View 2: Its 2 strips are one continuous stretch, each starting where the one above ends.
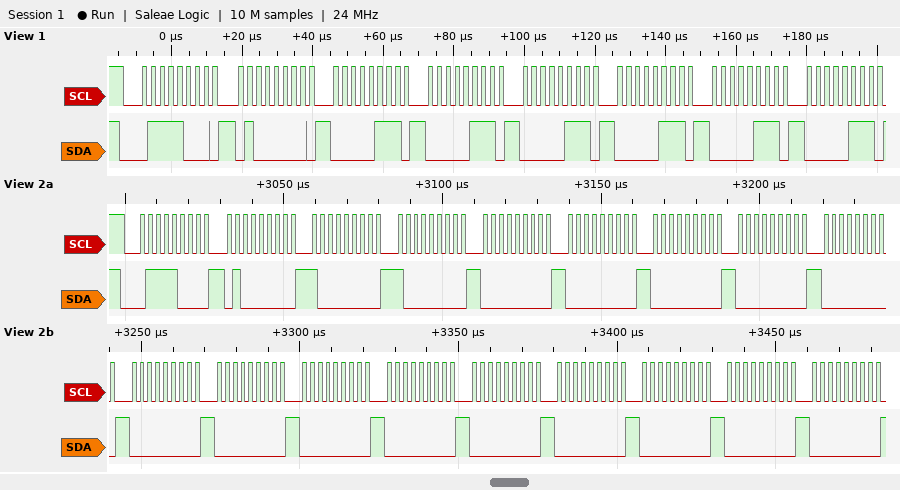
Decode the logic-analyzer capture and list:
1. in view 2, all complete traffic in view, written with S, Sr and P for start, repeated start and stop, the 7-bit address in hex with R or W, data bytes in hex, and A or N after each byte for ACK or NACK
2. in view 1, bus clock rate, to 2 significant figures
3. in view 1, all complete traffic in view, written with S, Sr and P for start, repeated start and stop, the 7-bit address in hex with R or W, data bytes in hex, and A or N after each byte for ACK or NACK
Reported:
S 3CW A 40 A 80 A 80 A 00 A 00 A 00 A 00 A 00 A 00 A 00 A 00 A 00 A 00 A 00 A 00 A 00 A 00 A
400 kHz
S 3CW A 40 A 07 A 07 A 07 A 07 A 07 A 07 A
